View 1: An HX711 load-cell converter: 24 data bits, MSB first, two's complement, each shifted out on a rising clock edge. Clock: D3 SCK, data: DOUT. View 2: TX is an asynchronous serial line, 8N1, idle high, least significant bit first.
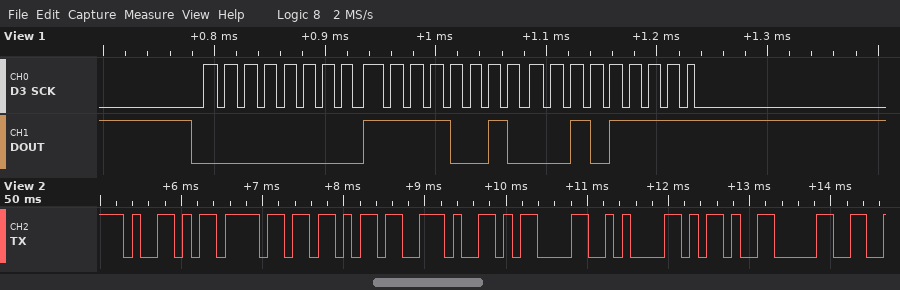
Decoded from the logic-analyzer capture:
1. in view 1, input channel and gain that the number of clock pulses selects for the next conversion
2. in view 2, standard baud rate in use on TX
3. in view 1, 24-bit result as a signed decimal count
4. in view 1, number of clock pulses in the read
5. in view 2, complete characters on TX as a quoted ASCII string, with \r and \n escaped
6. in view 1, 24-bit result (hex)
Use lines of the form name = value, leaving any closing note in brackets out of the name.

in view 1, input channel and gain that the number of clock pulses selects for the next conversion = channel A, gain 128
in view 2, standard baud rate in use on TX = 9600 baud
in view 1, 24-bit result as a signed decimal count = 61999
in view 1, number of clock pulses in the read = 25
in view 2, complete characters on TX as a quoted ASCII string, with \r and \n escaped = "Yok.\r\n-0"
in view 1, 24-bit result = 0x00F22F
